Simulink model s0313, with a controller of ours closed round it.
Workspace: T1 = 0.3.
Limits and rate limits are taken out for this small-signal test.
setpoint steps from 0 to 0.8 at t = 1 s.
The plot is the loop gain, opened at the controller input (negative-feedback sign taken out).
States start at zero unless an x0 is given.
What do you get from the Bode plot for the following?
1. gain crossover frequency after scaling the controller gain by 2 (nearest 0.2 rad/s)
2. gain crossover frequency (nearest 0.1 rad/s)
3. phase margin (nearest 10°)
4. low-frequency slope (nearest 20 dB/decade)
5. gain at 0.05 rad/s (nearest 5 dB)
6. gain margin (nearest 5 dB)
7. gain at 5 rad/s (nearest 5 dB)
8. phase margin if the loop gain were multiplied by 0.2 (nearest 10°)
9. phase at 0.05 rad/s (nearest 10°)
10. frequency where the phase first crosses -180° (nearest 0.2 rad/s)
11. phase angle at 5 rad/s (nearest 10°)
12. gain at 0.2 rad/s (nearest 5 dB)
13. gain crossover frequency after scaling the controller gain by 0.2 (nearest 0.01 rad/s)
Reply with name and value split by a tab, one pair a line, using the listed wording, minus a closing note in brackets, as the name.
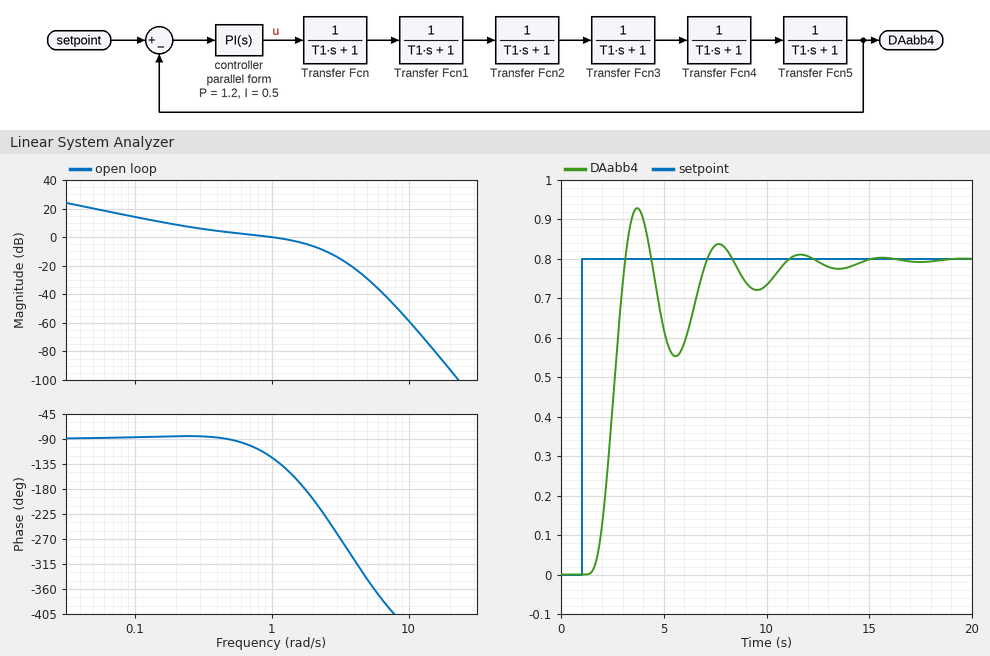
gain crossover frequency after scaling the controller gain by 2	2.0 rad/s
gain crossover frequency	1.0 rad/s
phase margin	60°
low-frequency slope	-20 dB/decade
gain at 0.05 rad/s	20 dB
gain margin	5 dB
gain at 5 rad/s	-30 dB
phase margin if the loop gain were multiplied by 0.2	90°
phase at 0.05 rad/s	-90°
frequency where the phase first crosses -180°	1.8 rad/s
phase angle at 5 rad/s	-340°
gain at 0.2 rad/s	10 dB
gain crossover frequency after scaling the controller gain by 0.2	0.10 rad/s
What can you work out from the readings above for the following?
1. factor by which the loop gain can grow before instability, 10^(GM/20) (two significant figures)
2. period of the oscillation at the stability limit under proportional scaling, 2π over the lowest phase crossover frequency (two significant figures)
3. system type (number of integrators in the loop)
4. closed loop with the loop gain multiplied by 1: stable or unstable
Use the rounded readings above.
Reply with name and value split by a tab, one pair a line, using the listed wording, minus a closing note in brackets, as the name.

factor by which the loop gain can grow before instability, 10^(GM/20)	1.8
period of the oscillation at the stability limit under proportional scaling, 2π over the lowest phase crossover frequency	3.5 s
system type	1
closed loop with the loop gain multiplied by 1: stable or unstable	stable
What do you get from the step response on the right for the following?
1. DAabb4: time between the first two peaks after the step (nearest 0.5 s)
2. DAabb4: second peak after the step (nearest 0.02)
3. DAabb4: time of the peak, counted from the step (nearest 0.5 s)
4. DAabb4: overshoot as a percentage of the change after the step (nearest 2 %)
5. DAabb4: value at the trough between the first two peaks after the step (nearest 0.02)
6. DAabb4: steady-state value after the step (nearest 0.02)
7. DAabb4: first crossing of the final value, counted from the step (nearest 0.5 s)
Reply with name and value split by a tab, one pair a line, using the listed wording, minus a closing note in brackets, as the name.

DAabb4: time between the first two peaks after the step	4.0 s
DAabb4: second peak after the step	0.84
DAabb4: time of the peak, counted from the step	2.5 s
DAabb4: overshoot as a percentage of the change after the step	16 %
DAabb4: value at the trough between the first two peaks after the step	0.56
DAabb4: steady-state value after the step	0.80
DAabb4: first crossing of the final value, counted from the step	2.0 s
